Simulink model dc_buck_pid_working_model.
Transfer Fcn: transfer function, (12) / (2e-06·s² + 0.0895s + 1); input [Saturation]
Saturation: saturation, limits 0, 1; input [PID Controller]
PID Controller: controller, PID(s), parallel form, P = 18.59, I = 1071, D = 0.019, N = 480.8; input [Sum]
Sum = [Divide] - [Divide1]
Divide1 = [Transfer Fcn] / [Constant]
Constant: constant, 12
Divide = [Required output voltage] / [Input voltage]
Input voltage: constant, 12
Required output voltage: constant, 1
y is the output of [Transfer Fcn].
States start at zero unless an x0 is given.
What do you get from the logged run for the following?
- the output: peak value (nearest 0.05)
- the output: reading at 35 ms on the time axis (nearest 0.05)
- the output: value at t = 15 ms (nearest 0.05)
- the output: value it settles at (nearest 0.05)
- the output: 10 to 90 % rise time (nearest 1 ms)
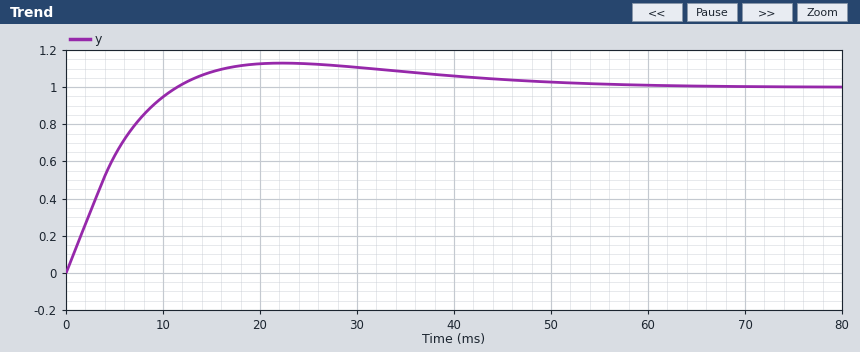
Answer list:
1.15
1.10
1.10
1.00
8 ms
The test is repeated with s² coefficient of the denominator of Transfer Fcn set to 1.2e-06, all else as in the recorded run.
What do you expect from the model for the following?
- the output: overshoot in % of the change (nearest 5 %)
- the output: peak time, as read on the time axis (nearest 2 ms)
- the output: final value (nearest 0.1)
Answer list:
15 %
22 ms
1.0
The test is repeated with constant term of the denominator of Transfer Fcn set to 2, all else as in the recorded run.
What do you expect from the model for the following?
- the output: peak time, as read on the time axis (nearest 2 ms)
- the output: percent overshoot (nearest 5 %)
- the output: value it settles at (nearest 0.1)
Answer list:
24 ms
10 %
1.0
